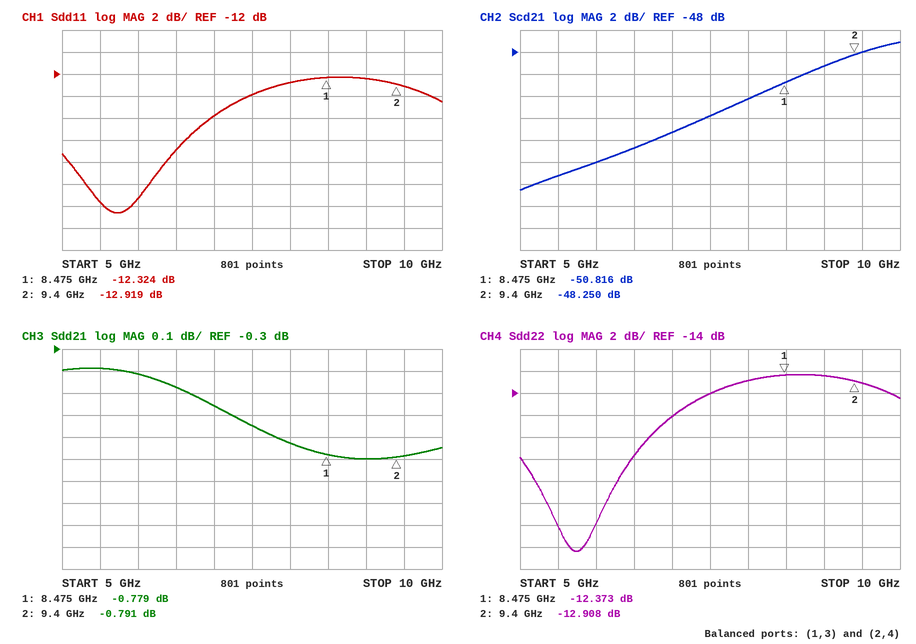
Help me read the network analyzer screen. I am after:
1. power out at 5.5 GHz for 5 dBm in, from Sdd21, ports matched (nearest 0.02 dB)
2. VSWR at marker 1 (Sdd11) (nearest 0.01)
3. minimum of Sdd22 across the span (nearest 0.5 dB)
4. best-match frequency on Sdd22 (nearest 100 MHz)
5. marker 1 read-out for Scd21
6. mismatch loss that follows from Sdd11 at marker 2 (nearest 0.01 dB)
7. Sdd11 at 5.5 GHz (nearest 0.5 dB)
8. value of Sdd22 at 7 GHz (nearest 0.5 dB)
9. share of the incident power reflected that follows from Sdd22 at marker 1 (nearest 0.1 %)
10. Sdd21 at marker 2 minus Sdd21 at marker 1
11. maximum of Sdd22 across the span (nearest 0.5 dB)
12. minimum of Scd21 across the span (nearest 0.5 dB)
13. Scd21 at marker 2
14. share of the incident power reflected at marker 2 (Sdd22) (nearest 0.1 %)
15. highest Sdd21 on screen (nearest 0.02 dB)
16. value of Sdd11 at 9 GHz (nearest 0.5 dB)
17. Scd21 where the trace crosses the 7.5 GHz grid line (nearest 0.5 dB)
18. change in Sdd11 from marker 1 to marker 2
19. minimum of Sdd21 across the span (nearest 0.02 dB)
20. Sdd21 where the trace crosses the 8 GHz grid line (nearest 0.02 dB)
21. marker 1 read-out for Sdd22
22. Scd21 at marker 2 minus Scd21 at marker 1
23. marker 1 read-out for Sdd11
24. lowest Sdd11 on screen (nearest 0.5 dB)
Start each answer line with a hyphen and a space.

- 4.62 dBm
- 1.64
- -28.5 dB
- 5.7 GHz
- -50.816 dB
- 0.23 dB
- -23.5 dB
- -16.0 dB
- 5.8 %
- -0.012 dB
- -12.5 dB
- -60.5 dB
- -48.250 dB
- 5.1 %
- -0.38 dB
- -12.5 dB
- -54.0 dB
- -0.595 dB
- -0.80 dB
- -0.72 dB
- -12.373 dB
- 2.566 dB
- -12.324 dB
- -24.5 dB
